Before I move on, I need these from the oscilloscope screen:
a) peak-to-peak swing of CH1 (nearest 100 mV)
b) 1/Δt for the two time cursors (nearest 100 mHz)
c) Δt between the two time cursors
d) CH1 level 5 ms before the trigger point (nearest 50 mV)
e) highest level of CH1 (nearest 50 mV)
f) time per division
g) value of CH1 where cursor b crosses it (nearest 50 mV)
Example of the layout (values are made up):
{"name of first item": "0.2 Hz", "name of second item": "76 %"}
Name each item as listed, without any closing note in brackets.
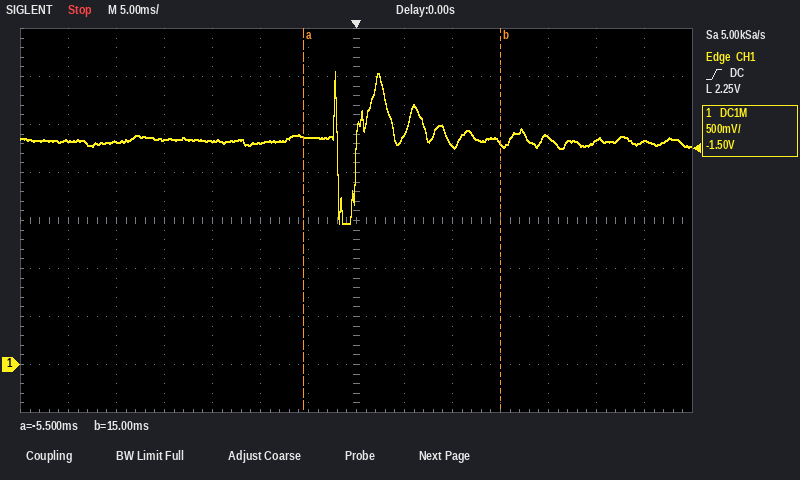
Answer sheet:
{"peak-to-peak swing of CH1": "1.60 V", "1/Δt for the two time cursors": "48.8 Hz", "Δt between the two time cursors": "20.5 ms", "CH1 level 5 ms before the trigger point": "2.35 V", "highest level of CH1": "3.05 V", "time per division": "5 ms", "value of CH1 where cursor b crosses it": "2.30 V"}
